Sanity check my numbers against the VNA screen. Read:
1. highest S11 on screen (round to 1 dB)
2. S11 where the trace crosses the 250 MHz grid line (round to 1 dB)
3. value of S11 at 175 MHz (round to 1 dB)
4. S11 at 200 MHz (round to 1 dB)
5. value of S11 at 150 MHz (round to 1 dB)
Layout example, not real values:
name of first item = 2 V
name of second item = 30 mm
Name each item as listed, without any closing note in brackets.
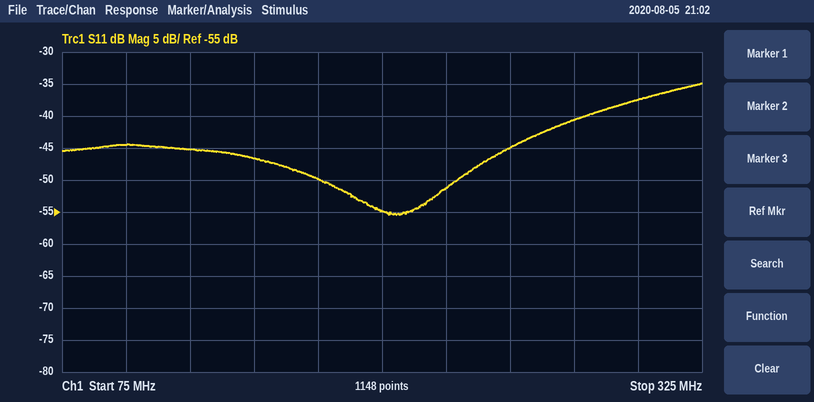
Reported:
highest S11 on screen = -35 dB
S11 where the trace crosses the 250 MHz grid line = -45 dB
value of S11 at 175 MHz = -50 dB
S11 at 200 MHz = -55 dB
value of S11 at 150 MHz = -47 dB
